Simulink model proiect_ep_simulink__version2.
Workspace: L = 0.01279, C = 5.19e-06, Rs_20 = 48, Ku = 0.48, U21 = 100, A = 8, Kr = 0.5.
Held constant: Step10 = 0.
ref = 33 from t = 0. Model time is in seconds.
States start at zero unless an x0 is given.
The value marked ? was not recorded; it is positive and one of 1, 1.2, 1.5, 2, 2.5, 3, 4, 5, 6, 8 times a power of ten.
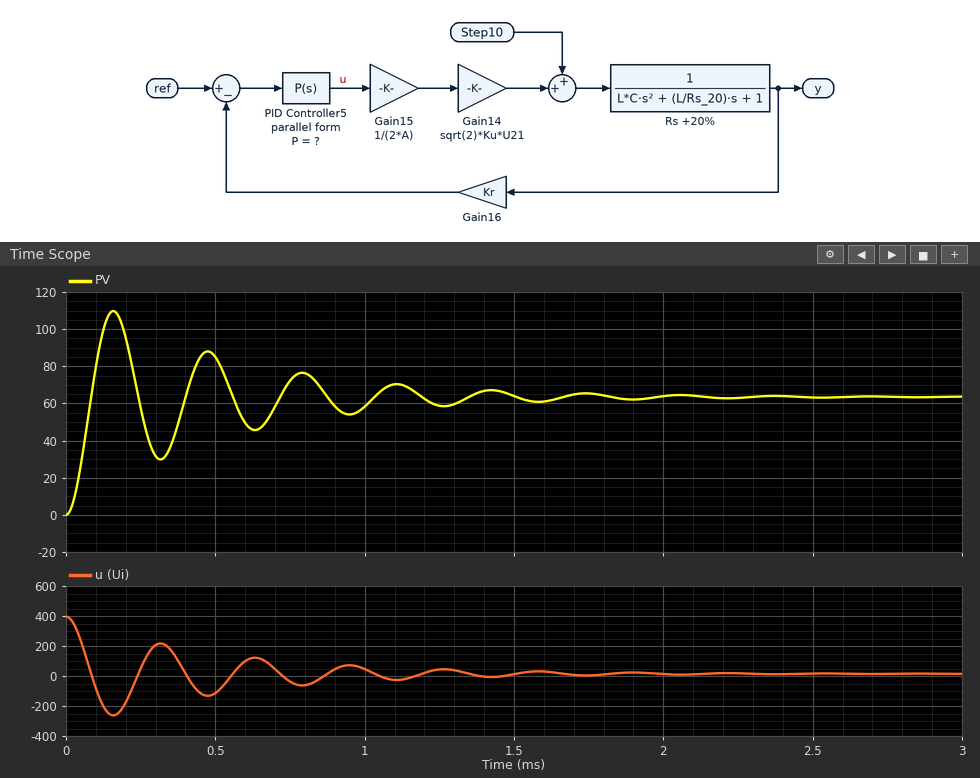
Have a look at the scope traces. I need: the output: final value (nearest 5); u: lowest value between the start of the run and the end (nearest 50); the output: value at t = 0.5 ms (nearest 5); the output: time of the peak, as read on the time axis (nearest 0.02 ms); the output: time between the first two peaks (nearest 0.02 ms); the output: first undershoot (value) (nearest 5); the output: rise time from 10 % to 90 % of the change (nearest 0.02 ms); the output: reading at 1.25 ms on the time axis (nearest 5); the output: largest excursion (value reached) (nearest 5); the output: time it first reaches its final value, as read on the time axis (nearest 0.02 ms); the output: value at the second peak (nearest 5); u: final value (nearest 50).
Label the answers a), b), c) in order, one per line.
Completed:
a) 65
b) -250
c) 85
d) 0.16 ms
e) 0.32 ms
f) 30
g) 0.06 ms
h) 60
i) 110
j) 0.08 ms
k) 90
l) 0
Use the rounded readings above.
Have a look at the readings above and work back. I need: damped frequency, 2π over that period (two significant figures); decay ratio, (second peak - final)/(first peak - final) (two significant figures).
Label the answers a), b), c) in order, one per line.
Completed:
a) 20 rad/ms
b) 0.56
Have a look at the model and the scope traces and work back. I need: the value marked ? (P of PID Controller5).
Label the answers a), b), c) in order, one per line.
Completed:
a) 12
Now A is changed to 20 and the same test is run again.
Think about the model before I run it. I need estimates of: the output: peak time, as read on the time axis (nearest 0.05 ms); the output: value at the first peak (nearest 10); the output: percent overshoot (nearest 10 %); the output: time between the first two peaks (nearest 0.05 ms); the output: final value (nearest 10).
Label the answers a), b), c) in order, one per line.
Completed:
a) 0.25 ms
b) 100
c) 60 %
d) 0.50 ms
e) 60
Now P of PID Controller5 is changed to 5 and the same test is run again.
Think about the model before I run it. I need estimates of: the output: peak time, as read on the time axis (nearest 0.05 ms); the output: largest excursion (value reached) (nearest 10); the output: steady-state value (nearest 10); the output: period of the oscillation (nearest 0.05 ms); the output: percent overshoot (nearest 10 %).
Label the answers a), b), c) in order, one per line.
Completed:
a) 0.25 ms
b) 100
c) 60
d) 0.50 ms
e) 60 %
